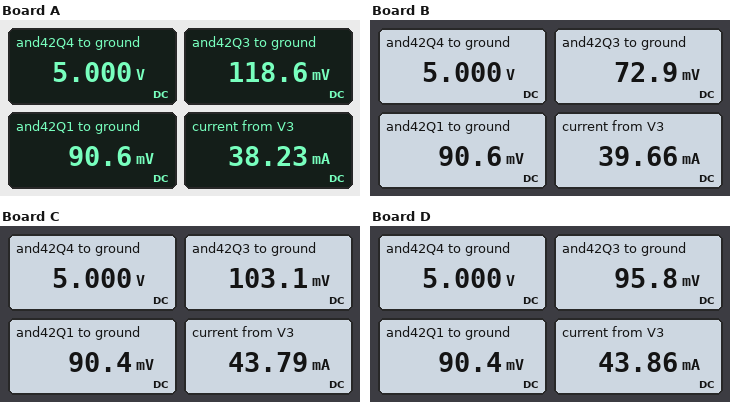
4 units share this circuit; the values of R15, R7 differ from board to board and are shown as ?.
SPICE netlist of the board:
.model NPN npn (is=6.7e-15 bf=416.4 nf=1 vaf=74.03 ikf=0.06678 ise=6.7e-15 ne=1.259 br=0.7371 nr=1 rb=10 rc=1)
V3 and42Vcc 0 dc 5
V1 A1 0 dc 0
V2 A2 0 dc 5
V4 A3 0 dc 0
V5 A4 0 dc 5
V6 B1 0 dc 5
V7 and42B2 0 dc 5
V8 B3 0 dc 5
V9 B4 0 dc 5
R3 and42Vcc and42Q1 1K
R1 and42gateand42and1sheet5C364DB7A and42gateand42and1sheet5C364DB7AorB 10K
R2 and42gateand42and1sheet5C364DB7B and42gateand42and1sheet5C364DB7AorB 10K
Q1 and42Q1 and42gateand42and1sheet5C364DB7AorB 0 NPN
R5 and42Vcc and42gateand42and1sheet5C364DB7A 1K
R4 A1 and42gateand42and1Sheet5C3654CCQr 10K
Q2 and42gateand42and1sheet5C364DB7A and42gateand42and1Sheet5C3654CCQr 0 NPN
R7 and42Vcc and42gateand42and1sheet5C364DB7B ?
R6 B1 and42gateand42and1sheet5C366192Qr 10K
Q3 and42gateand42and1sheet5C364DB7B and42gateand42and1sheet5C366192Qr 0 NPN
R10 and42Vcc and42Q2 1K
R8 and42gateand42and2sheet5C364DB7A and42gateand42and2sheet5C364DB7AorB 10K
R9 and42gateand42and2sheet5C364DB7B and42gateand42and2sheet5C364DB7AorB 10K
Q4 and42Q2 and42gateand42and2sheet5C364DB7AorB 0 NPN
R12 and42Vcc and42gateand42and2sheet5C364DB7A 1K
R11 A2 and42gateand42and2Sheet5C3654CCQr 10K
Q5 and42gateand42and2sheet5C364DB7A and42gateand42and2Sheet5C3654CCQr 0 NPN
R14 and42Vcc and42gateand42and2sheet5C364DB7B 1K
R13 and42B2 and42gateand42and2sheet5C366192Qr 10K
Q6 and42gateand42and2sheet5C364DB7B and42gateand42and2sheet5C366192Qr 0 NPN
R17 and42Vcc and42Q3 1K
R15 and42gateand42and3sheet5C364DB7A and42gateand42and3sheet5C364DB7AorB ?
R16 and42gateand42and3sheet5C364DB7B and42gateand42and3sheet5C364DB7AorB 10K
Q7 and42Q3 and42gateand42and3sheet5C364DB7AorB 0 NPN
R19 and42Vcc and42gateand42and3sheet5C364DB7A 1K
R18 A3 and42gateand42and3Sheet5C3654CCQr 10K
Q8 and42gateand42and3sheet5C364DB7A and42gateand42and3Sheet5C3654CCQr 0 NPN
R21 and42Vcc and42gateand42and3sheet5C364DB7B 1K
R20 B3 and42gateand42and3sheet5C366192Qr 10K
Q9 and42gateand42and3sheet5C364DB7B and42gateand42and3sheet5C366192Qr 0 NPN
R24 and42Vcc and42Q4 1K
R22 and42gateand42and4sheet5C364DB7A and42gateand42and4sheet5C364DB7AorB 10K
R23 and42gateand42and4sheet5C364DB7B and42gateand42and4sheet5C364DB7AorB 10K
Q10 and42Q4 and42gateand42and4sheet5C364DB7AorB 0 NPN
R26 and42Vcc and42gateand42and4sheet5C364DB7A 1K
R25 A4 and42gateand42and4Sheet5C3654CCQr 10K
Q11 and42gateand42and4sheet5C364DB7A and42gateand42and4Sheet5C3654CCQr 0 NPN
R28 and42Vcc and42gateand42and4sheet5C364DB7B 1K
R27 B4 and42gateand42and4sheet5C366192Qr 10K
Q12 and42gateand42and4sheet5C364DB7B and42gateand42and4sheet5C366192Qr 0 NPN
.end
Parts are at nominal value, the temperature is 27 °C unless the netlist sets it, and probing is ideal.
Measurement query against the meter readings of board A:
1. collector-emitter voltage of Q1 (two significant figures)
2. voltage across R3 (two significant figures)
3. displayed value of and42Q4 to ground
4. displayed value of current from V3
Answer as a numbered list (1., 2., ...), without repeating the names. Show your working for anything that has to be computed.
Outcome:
1. 90.6 mV = 91 mV
2. 5 V - 90.6 mV = 4.9 V
3. 5.000 V
4. 38.23 mA
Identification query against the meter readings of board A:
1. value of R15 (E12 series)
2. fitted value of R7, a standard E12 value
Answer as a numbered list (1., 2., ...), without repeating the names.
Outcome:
1. 22 kΩ
2. 1.5 kΩ
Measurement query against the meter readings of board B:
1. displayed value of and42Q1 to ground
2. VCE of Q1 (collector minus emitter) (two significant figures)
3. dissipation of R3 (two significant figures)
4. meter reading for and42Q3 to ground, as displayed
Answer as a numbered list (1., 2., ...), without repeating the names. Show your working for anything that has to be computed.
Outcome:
1. 90.6 mV
2. 90.6 mV = 91 mV
3. (5 V - 90.6 mV)^2 / 1 kΩ = 24 mW
4. 72.9 mV
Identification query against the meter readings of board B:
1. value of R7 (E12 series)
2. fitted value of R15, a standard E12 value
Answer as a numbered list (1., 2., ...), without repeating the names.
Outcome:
1. 1.2 kΩ
2. 4.7 kΩ
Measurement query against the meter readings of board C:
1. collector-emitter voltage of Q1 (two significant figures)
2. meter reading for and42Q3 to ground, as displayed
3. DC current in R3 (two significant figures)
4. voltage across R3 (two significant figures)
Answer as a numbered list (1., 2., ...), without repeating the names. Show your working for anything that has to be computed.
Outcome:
1. 90.4 mV = 90 mV
2. 103.1 mV
3. (5 V - 90.4 mV) / 1 kΩ = 4.9 mA
4. 5 V - 90.4 mV = 4.9 V
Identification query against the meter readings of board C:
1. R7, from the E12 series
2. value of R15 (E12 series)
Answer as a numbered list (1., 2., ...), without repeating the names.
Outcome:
1. 560 Ω
2. 15 kΩ
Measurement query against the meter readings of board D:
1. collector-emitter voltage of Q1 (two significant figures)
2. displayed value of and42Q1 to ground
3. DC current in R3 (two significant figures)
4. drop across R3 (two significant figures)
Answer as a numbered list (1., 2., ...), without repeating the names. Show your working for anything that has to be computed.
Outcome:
1. 90.4 mV = 90 mV
2. 90.4 mV
3. (5 V - 90.4 mV) / 1 kΩ = 4.9 mA
4. 5 V - 90.4 mV = 4.9 V
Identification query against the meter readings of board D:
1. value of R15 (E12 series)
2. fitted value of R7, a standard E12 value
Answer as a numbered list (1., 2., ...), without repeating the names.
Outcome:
1. 12 kΩ
2. 560 Ω
